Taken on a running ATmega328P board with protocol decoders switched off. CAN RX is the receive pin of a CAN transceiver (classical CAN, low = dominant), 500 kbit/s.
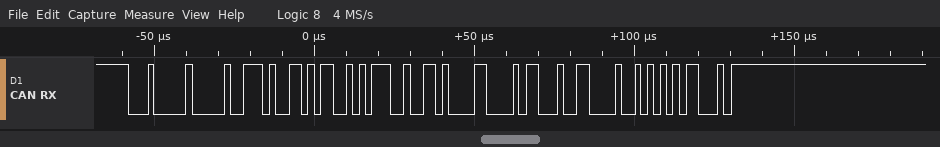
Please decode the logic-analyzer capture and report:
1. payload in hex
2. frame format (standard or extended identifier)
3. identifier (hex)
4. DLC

4D 65 72 68 61 62 61
standard
0x100
7
